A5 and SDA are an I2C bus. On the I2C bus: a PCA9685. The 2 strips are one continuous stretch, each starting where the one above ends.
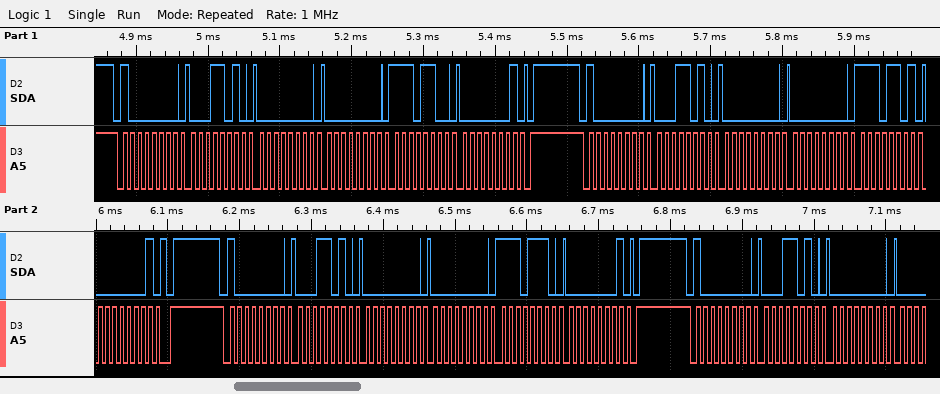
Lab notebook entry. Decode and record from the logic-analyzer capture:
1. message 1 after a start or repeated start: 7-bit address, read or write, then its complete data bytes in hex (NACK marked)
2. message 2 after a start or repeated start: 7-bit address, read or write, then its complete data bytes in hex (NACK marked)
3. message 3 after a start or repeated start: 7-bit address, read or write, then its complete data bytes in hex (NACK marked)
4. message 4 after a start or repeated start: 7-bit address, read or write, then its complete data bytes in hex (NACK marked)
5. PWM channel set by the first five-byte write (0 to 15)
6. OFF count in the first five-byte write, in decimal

0x40 write: 1A 00 00 EC 01
0x40 write: 1A 00 00 ED 01
0x40 write: 1A 00 00 EE 01
0x40 write: 1A 00
5
492
